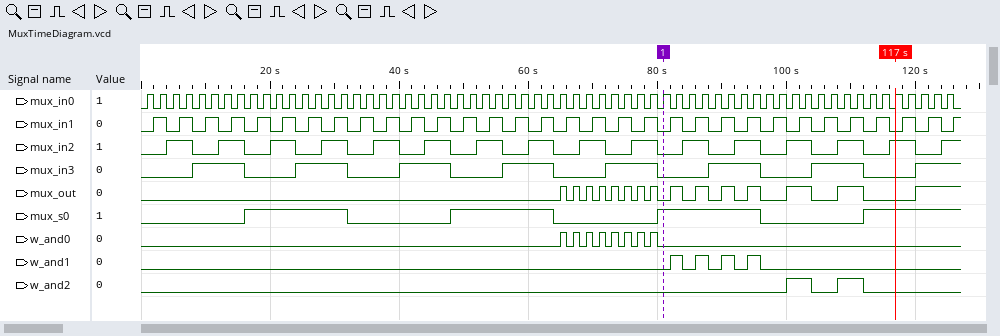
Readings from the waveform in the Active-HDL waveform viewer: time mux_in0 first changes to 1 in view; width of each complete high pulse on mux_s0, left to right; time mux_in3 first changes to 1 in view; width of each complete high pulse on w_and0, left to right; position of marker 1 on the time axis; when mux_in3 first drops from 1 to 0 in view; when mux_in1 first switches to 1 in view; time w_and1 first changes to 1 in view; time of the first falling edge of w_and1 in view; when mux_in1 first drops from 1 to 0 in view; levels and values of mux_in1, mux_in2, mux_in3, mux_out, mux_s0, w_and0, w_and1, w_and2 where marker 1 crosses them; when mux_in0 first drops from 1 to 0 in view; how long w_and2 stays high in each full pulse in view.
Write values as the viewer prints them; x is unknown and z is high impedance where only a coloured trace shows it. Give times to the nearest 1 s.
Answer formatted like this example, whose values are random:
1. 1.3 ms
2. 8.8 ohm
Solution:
1. 1 s
2. 16 s, 16 s, 16 s
3. 8 s
4. 1 s, 1 s, 1 s, 1 s, 1 s, 1 s, 1 s, 1 s
5. 81 s
6. 16 s
7. 2 s
8. 82 s
9. 84 s
10. 4 s
11. mux_in1=0, mux_in2=0, mux_in3=0, mux_out=0, mux_s0=1, w_and0=0, w_and1=0, w_and2=0
12. 2 s
13. 4 s, 4 s
